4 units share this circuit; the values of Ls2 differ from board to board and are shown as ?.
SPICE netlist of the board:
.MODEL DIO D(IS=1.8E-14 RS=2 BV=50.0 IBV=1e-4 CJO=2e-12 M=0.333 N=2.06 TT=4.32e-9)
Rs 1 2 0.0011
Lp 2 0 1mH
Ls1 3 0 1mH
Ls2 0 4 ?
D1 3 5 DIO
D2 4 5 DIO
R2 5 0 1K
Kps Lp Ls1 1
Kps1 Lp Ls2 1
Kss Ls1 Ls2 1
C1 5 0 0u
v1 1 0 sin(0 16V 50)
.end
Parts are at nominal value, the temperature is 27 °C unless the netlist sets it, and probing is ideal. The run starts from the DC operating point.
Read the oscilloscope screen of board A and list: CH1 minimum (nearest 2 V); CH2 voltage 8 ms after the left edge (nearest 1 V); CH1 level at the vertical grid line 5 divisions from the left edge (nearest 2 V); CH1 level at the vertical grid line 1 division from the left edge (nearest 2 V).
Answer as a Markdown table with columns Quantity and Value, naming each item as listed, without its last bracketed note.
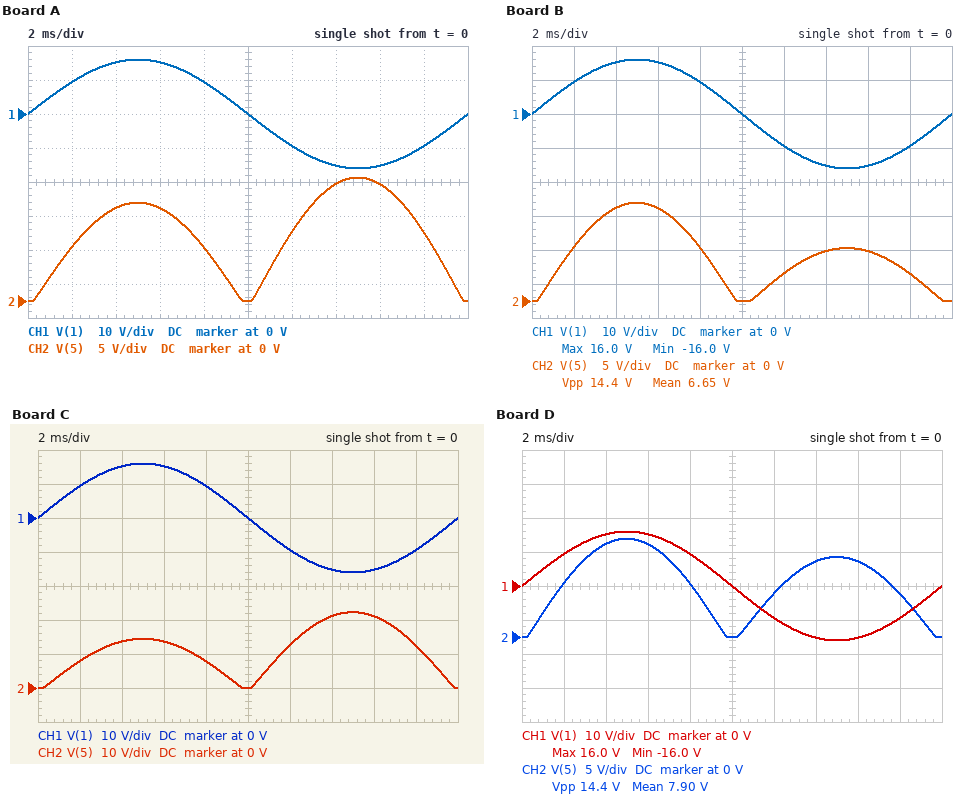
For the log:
| Quantity | Value |
|---|---|
| CH1 minimum | -16 V |
| CH2 voltage 8 ms after the left edge | 8 V |
| CH1 level at the vertical grid line 5 divisions from the left edge | 0 V |
| CH1 level at the vertical grid line 1 division from the left edge | 10 V |
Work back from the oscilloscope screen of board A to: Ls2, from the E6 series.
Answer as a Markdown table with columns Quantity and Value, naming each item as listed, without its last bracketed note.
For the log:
| Quantity | Value |
|---|---|
| Ls2, from the E6 series | 1.5 mH |
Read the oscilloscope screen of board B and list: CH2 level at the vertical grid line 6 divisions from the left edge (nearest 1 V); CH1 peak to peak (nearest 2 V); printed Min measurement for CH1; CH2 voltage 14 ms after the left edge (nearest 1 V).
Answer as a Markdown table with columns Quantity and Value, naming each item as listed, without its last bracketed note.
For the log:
| Quantity | Value |
|---|---|
| CH2 level at the vertical grid line 6 divisions from the left edge | 4 V |
| CH1 peak to peak | 32 V |
| printed Min measurement for CH1 | -16.0 V |
| CH2 voltage 14 ms after the left edge | 7 V |
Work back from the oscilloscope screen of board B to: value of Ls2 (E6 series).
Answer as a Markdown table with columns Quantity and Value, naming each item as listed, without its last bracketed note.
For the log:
| Quantity | Value |
|---|---|
| value of Ls2 | 330 µH |
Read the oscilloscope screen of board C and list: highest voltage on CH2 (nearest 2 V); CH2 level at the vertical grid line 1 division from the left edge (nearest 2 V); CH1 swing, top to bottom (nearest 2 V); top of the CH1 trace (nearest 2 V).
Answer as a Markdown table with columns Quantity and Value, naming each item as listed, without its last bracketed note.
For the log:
| Quantity | Value |
|---|---|
| highest voltage on CH2 | 22 V |
| CH2 level at the vertical grid line 1 division from the left edge | 8 V |
| CH1 swing, top to bottom | 32 V |
| top of the CH1 trace | 16 V |
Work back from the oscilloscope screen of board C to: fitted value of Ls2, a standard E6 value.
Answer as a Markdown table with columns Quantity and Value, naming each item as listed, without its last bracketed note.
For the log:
| Quantity | Value |
|---|---|
| fitted value of Ls2, a standard E6 value | 2.2 mH |
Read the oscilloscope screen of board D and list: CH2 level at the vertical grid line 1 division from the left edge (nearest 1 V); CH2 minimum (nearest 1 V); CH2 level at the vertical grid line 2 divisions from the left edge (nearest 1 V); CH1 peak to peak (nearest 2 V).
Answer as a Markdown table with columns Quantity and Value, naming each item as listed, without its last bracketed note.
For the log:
| Quantity | Value |
|---|---|
| CH2 level at the vertical grid line 1 division from the left edge | 8 V |
| CH2 minimum | 0 V |
| CH2 level at the vertical grid line 2 divisions from the left edge | 14 V |
| CH1 peak to peak | 32 V |
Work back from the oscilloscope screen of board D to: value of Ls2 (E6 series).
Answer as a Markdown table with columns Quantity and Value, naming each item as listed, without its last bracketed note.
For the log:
| Quantity | Value |
|---|---|
| value of Ls2 | 680 µH |
